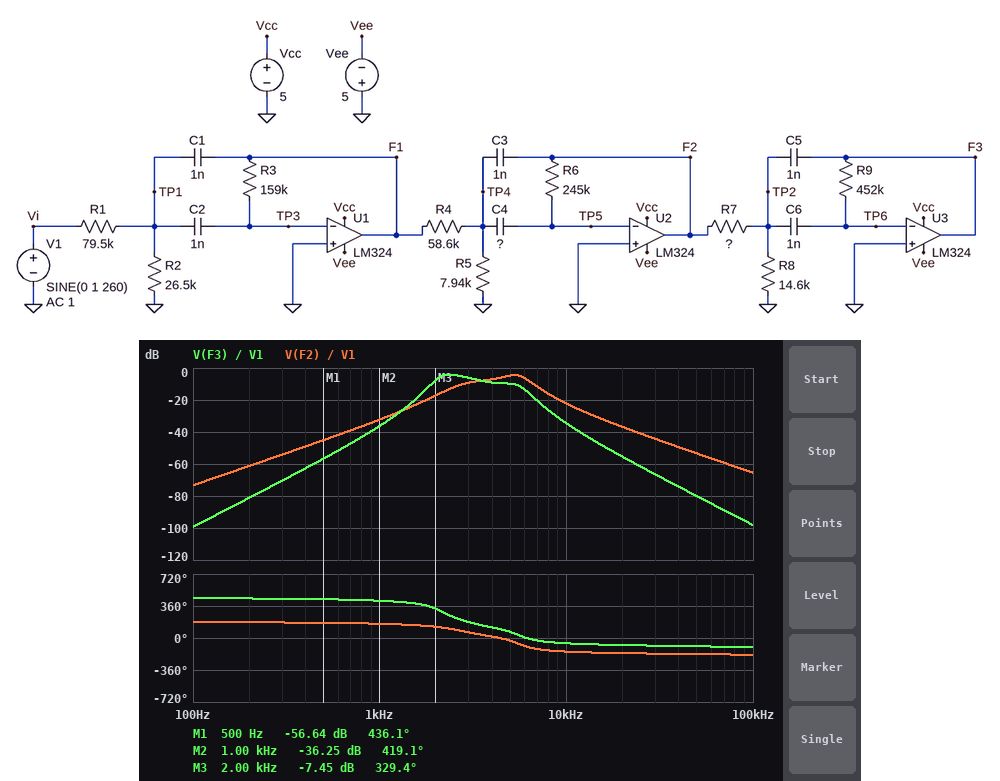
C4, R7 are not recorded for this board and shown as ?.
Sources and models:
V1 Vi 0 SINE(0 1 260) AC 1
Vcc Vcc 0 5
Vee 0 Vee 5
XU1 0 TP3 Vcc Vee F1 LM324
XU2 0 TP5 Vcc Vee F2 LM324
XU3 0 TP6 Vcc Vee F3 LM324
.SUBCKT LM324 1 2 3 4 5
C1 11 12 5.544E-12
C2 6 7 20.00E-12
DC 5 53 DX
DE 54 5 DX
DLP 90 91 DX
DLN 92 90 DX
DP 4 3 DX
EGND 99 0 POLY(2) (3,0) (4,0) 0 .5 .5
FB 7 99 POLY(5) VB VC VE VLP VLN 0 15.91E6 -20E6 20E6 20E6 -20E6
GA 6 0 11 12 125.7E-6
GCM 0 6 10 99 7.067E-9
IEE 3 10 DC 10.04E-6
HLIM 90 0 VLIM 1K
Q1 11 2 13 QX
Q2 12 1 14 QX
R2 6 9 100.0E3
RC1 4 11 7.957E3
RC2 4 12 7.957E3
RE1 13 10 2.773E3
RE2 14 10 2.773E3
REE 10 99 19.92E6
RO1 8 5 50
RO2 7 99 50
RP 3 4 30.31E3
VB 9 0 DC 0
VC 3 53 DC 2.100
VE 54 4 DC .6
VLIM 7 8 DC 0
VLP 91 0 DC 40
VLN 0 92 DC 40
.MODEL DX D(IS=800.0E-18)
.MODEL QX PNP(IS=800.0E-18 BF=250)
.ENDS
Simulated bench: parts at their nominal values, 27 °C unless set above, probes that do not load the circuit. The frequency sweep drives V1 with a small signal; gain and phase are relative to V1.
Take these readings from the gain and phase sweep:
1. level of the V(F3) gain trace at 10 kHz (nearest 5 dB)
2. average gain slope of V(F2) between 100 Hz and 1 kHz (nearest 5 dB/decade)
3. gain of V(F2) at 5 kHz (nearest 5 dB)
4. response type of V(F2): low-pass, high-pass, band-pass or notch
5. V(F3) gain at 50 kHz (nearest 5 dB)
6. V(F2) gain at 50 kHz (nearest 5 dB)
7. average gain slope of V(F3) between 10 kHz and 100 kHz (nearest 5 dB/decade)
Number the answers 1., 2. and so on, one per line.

1. -35 dB
2. 40 dB/decade
3. -5 dB
4. band-pass
5. -80 dB
6. -55 dB
7. -65 dB/decade
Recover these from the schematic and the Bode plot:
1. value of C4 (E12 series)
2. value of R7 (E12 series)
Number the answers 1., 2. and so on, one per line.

1. 470 pF
2. 68 kΩ
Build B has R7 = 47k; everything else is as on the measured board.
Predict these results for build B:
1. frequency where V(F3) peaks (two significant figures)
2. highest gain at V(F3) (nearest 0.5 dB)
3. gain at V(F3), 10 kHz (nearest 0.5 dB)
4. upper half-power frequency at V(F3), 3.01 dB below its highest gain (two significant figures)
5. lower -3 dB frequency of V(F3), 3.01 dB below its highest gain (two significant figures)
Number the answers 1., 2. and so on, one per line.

1. 2.4 kHz
2. 0 dB
3. -31.5 dB
4. 3.2 kHz
5. 2.1 kHz
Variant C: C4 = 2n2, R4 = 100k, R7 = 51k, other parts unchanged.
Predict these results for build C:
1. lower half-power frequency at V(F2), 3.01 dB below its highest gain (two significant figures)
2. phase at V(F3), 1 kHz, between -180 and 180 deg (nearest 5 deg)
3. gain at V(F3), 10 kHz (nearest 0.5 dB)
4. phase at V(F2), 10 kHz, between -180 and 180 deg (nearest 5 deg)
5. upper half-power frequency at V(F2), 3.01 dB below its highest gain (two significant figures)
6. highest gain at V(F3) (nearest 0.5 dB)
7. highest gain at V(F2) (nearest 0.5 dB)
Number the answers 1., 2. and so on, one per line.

1. 2.2 kHz
2. 55 deg
3. -39.0 dB
4. -165 deg
5. 3.0 kHz
6. 15.5 dB
7. 4.0 dB
